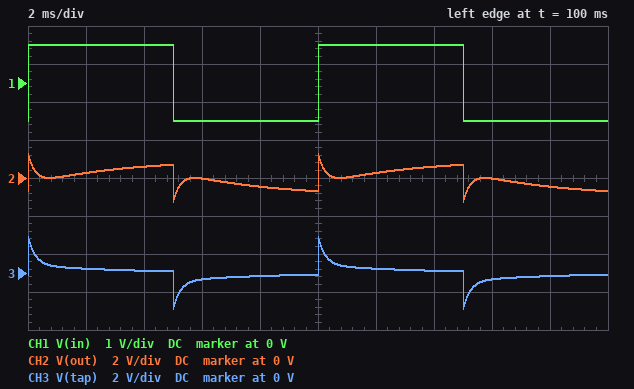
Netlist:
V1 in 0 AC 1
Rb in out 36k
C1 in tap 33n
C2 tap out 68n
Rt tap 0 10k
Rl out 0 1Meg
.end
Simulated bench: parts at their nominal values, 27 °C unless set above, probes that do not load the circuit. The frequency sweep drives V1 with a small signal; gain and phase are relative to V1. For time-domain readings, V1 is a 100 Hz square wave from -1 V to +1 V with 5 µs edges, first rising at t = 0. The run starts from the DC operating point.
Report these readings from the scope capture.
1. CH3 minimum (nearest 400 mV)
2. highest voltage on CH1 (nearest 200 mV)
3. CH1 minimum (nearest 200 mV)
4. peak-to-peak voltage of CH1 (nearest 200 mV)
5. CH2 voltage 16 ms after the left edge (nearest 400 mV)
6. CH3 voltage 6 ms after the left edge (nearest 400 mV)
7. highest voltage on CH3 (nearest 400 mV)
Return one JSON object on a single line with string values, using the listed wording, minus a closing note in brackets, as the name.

{"CH3 minimum": "-2.0 V", "highest voltage on CH1": "1.0 V", "CH1 minimum": "-1.0 V", "peak-to-peak voltage of CH1": "2.0 V", "CH2 voltage 16 ms after the left edge": "0 V", "CH3 voltage 6 ms after the left edge": "-400 mV", "highest voltage on CH3": "2.0 V"}
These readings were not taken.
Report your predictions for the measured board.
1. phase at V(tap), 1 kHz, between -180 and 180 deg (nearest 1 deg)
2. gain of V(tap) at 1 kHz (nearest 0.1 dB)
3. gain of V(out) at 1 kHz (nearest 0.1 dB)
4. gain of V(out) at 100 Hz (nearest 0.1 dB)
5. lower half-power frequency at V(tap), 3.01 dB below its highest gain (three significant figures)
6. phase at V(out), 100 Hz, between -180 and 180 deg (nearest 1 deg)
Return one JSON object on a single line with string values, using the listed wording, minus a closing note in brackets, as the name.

{"phase at V(tap), 1 kHz, between -180 and 180 deg": "24 deg", "gain of V(tap) at 1 kHz": "-1.3 dB", "gain of V(out) at 1 kHz": "-1.6 dB", "gain of V(out) at 100 Hz": "-7.9 dB", "lower half-power frequency at V(tap), 3.01 dB below its highest gain": "575 Hz", "phase at V(out), 100 Hz, between -180 and 180 deg": "-29 deg"}
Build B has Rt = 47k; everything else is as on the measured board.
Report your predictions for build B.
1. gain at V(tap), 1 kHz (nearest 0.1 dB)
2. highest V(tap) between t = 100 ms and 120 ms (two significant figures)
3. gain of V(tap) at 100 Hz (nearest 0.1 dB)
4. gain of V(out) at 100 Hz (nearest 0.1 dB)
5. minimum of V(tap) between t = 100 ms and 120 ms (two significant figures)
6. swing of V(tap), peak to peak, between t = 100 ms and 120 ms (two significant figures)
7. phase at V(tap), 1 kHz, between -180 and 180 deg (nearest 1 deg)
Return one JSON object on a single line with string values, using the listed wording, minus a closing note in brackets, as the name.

{"gain at V(tap), 1 kHz": "-0.2 dB", "highest V(tap) between t = 100 ms and 120 ms": "1.6 V", "gain of V(tap) at 100 Hz": "-2.8 dB", "gain of V(out) at 100 Hz": "-3.7 dB", "minimum of V(tap) between t = 100 ms and 120 ms": "-1.6 V", "swing of V(tap), peak to peak, between t = 100 ms and 120 ms": "3.1 V", "phase at V(tap), 1 kHz, between -180 and 180 deg": "6 deg"}
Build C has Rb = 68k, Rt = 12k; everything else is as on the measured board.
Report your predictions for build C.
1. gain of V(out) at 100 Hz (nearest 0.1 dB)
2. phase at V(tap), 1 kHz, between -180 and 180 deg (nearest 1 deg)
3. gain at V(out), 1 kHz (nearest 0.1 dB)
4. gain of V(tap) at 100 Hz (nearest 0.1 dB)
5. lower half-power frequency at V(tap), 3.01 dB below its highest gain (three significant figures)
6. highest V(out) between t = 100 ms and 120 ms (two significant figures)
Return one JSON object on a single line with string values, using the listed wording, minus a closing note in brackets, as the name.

{"gain of V(out) at 100 Hz": "-13.3 dB", "phase at V(tap), 1 kHz, between -180 and 180 deg": "21 deg", "gain at V(out), 1 kHz": "-1.0 dB", "gain of V(tap) at 100 Hz": "-10.9 dB", "lower half-power frequency at V(tap), 3.01 dB below its highest gain": "461 Hz", "highest V(out) between t = 100 ms and 120 ms": "1.5 V"}
